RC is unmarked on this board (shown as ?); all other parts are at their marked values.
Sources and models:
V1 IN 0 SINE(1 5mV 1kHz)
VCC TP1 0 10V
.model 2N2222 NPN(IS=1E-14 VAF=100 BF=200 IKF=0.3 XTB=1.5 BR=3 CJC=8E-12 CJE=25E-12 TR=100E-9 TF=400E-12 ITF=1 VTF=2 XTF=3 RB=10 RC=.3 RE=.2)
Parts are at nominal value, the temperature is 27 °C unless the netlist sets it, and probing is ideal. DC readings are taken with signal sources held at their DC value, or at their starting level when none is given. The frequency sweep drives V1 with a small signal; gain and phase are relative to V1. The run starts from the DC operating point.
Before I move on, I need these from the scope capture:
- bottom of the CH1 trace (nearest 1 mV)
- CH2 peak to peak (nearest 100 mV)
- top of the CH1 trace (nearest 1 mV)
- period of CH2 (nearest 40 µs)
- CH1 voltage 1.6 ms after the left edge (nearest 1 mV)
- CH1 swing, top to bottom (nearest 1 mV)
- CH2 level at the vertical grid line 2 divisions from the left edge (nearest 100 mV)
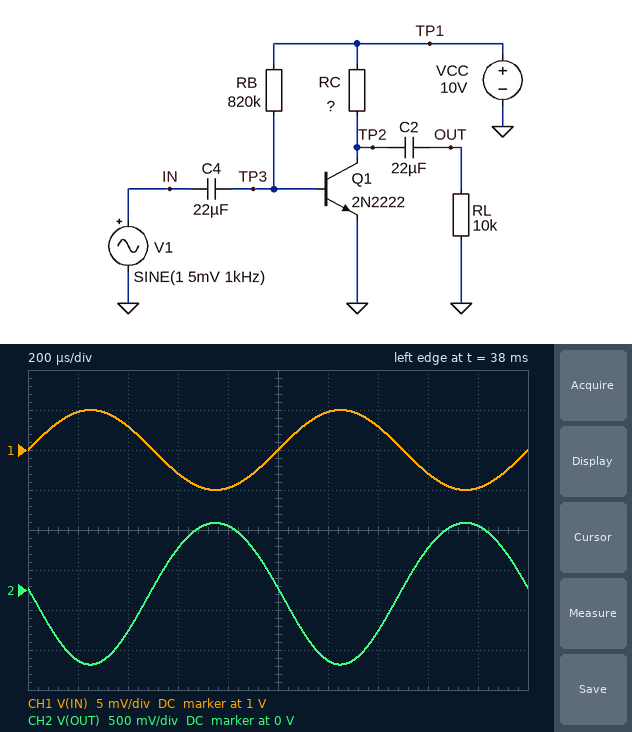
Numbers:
995 mV
1.8 V
1.005 V
1.00 ms
997 mV
10 mV
-500 mV
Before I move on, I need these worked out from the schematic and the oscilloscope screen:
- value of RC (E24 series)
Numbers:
2.7 kΩ
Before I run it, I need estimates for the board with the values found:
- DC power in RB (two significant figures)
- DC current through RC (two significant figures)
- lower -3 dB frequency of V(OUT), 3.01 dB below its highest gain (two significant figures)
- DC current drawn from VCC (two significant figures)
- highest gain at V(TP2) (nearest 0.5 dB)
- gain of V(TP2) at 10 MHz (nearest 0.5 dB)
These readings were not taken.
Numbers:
110 µW
2.3 mA
3.2 Hz
2.3 mA
45.0 dB
41.5 dB
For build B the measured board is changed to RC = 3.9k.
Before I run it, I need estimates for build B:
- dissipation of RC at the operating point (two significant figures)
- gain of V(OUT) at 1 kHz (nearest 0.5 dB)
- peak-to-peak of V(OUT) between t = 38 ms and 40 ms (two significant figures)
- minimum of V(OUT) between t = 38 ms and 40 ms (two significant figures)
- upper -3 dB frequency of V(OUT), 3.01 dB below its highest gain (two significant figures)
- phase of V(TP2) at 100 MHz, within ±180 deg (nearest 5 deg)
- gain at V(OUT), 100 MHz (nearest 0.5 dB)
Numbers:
20 mW
47.0 dB
2.2 V
-1.0 V
4.7 MHz
75 deg
20.5 dB
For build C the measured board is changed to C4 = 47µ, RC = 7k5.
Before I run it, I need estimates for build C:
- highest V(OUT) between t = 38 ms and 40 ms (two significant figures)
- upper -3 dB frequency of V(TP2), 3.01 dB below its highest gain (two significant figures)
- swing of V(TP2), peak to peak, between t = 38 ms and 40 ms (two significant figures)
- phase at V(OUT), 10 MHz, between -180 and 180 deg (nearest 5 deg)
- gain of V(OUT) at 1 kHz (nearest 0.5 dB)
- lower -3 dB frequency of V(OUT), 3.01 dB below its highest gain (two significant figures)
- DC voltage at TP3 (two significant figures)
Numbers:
1.3 V
1.7 MHz
1.4 V
95 deg
33.5 dB
30 Hz
660 mV
